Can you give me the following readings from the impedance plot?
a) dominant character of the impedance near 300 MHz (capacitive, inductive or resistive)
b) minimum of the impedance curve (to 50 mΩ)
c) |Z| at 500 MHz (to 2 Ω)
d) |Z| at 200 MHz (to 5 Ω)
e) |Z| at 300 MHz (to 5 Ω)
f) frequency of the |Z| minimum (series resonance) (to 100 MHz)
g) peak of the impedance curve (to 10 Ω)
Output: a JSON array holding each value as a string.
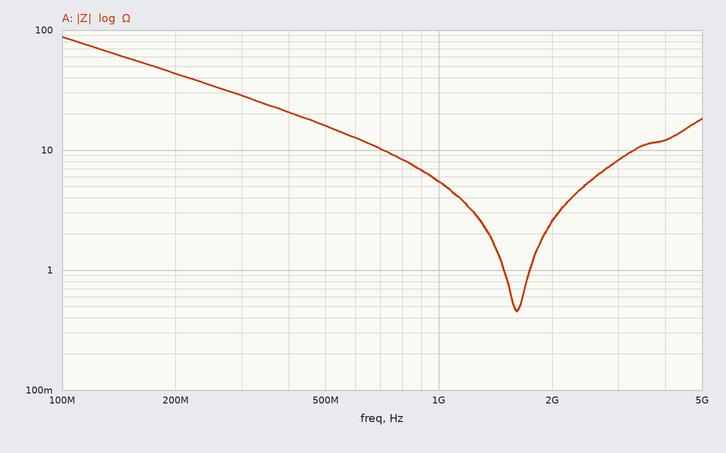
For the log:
["capacitive", "450 mΩ", "16 Ω", "45 Ω", "30 Ω", "1.6 GHz", "90 Ω"]
